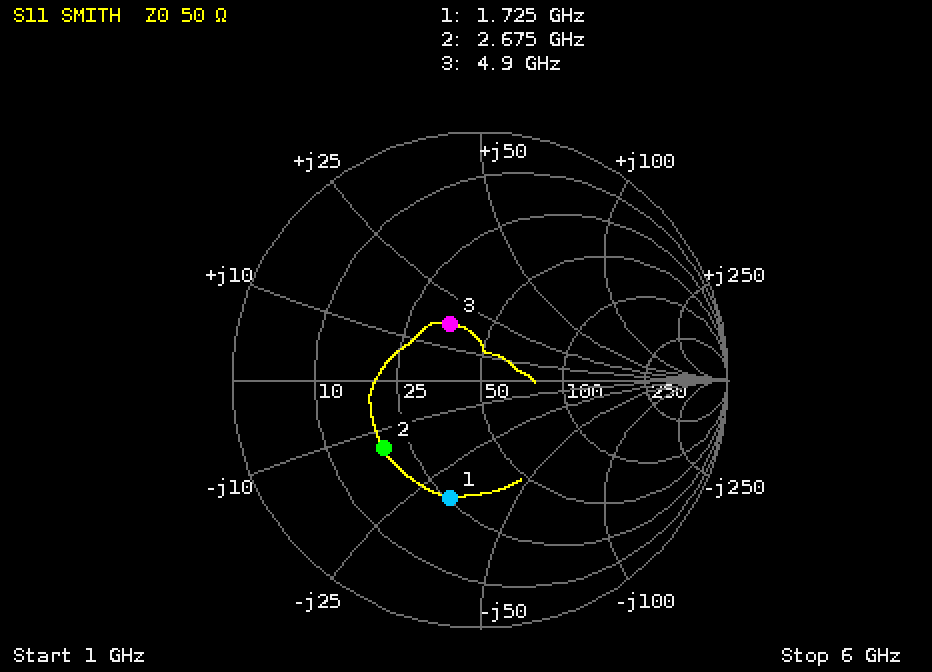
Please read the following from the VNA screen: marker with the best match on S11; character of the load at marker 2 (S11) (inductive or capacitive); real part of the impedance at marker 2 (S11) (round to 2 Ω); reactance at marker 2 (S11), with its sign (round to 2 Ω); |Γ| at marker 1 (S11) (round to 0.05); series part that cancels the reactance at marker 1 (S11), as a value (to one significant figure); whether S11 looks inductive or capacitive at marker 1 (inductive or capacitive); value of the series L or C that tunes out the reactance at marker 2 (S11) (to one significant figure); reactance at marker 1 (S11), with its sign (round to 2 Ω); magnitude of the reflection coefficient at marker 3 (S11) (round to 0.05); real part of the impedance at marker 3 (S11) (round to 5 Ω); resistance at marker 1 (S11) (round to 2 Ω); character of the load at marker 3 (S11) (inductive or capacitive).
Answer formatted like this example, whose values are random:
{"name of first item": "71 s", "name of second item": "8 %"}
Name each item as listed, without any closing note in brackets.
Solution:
{"marker with the best match on S11": "marker 3", "character of the load at marker 2 (S11)": "capacitive", "real part of the impedance at marker 2 (S11)": "20 Ω", "reactance at marker 2 (S11), with its sign": "-14 Ω", "|Γ| at marker 1 (S11)": "0.50", "series part that cancels the reactance at marker 1 (S11), as a value": "3 nH", "whether S11 looks inductive or capacitive at marker 1": "capacitive", "value of the series L or C that tunes out the reactance at marker 2 (S11)": "800 pH", "reactance at marker 1 (S11), with its sign": "-32 Ω", "magnitude of the reflection coefficient at marker 3 (S11)": "0.25", "real part of the impedance at marker 3 (S11)": "35 Ω", "resistance at marker 1 (S11)": "26 Ω", "character of the load at marker 3 (S11)": "inductive"}
